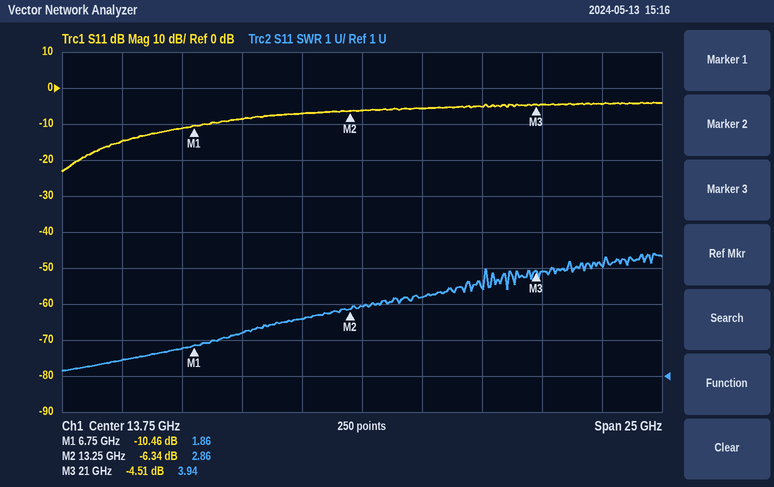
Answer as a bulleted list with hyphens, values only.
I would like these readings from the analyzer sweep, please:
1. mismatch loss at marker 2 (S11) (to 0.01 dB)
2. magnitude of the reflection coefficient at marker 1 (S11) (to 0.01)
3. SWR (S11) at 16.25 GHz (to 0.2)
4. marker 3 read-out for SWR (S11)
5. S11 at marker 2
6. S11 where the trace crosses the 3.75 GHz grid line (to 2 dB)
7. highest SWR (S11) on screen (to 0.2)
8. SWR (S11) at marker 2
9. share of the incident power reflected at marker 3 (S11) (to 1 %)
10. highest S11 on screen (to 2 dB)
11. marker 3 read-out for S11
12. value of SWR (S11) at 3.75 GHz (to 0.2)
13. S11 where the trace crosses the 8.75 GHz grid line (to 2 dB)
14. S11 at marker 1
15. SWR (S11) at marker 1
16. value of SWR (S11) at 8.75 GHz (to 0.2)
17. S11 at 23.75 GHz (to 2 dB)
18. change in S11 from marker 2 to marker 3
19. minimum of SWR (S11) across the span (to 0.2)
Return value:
- 1.15 dB
- 0.30
- 3.2
- 3.94
- -6.34 dB
- -14 dB
- 4.4
- 2.86
- 35 %
- -4 dB
- -4.51 dB
- 1.4
- -8 dB
- -10.46 dB
- 1.86
- 2.2
- -4 dB
- 1.83 dB
- 1.2
